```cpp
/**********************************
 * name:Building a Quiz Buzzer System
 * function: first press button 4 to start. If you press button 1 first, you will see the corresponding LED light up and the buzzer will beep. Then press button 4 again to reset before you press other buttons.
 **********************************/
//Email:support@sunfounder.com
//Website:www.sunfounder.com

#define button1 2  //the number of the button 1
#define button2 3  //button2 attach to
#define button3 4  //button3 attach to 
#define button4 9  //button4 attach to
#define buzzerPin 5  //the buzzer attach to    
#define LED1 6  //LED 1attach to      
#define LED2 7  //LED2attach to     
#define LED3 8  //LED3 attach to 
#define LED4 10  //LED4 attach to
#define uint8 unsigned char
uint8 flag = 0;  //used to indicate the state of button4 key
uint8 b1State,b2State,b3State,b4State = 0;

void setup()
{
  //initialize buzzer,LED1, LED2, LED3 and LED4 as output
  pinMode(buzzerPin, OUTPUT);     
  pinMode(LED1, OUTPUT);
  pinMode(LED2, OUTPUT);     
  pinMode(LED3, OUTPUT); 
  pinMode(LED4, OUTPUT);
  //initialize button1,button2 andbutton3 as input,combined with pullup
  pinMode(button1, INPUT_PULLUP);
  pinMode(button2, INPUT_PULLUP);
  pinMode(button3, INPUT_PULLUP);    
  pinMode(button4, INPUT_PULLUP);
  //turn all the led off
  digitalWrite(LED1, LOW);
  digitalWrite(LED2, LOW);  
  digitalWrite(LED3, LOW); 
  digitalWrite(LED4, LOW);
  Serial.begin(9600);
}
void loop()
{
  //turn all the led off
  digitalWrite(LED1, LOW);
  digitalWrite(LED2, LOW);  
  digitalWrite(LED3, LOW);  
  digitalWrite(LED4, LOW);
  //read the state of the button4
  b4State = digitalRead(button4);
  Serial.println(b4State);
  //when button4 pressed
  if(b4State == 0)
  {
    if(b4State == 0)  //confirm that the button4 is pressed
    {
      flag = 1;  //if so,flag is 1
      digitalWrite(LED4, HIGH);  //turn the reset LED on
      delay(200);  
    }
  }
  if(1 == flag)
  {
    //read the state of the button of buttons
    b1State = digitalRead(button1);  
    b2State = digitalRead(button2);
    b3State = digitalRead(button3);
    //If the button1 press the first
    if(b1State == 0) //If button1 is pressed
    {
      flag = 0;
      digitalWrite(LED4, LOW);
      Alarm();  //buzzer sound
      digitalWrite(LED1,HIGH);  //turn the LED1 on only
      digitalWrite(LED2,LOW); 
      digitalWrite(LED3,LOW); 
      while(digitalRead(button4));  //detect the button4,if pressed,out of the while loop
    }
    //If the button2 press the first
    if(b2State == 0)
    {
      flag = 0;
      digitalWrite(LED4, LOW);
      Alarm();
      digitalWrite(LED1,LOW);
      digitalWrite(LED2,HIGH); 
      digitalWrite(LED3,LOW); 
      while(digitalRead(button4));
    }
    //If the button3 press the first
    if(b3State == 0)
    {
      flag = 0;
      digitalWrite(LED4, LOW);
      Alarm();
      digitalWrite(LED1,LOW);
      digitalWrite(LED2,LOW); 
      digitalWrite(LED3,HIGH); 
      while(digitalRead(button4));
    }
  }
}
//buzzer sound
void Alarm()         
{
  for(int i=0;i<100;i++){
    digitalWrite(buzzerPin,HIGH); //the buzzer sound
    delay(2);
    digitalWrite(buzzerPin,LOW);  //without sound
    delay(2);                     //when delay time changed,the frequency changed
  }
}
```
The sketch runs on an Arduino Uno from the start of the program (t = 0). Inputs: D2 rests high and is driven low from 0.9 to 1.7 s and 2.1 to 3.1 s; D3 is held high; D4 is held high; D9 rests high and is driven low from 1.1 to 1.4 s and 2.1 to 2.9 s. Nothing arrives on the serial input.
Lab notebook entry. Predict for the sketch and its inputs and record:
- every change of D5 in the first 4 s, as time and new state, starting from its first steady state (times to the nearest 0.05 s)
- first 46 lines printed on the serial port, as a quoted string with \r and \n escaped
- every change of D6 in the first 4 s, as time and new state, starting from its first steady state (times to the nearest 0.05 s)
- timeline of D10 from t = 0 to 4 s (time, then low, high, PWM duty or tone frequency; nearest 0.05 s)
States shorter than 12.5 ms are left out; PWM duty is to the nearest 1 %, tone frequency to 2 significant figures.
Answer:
0 s low; 1.3 s tone 250 Hz; 1.7 s low; 2.3 s tone 250 Hz; 2.7 s low; 2.9 s tone 250 Hz; 3.3 s low
"1\r\n1\r\n1\r\n1\r\n1\r\n1\r\n1\r\n1\r\n1\r\n1\r\n1\r\n1\r\n1\r\n1\r\n1\r\n1\r\n1\r\n1\r\n1\r\n1\r\n1\r\n1\r\n1\r\n1\r\n1\r\n1\r\n1\r\n1\r\n1\r\n1\r\n1\r\n1\r\n1\r\n1\r\n1\r\n1\r\n1\r\n1\r\n1\r\n1\r\n1\r\n1\r\n1\r\n1\r\n1\r\n1\r\n"
0 s low; 1.7 s high; 2.1 s low; 3.3 s high
0 s low; 1.1 s high; 1.3 s low; 2.1 s high; 2.3 s low; 2.7 s high; 2.9 s low
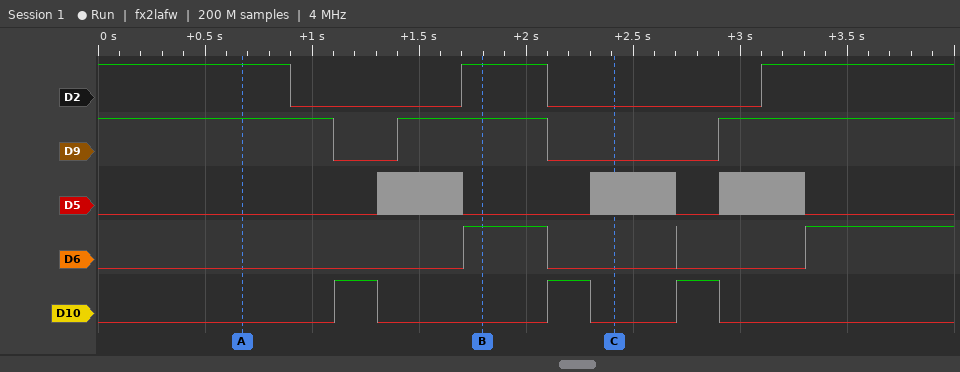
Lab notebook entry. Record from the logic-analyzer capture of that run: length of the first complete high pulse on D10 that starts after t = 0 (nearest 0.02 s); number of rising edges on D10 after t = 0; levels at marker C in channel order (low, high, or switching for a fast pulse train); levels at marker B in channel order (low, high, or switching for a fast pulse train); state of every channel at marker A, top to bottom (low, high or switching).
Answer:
0.20 s
3
D2 low, D9 low, D5 switching, D6 low, D10 low
D2 high, D9 high, D5 low, D6 high, D10 low
D2 high, D9 high, D5 low, D6 low, D10 low
